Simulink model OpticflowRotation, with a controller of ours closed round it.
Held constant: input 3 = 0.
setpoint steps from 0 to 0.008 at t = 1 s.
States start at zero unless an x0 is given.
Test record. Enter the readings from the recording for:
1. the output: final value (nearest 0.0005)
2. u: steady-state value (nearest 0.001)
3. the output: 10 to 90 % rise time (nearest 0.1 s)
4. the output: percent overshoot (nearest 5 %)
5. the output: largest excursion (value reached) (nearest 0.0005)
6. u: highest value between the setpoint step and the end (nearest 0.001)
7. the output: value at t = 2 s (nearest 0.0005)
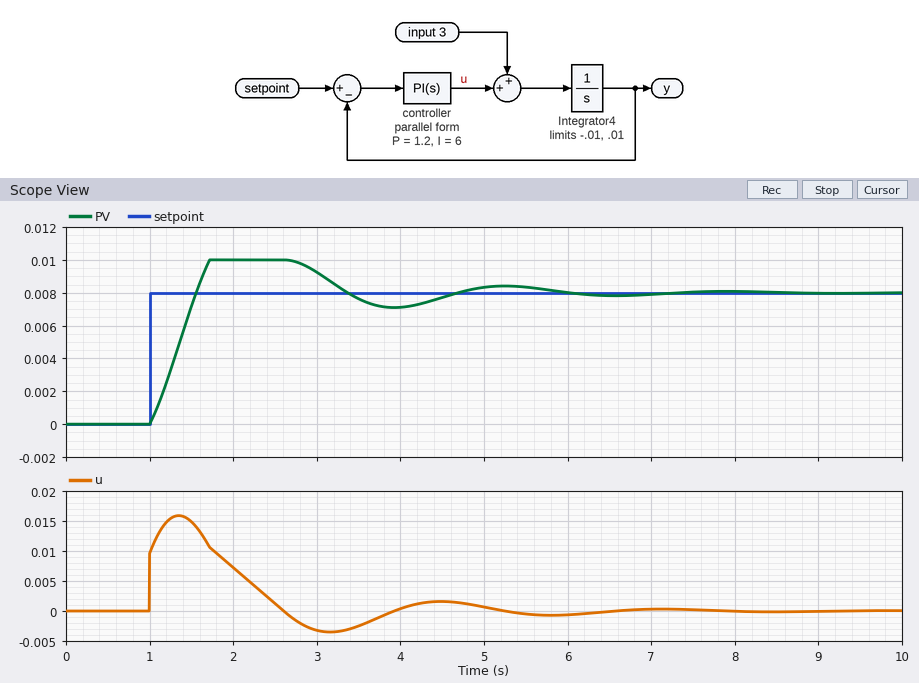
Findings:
0.0080
0.000
0.4 s
25 %
0.0100
0.016
0.0100
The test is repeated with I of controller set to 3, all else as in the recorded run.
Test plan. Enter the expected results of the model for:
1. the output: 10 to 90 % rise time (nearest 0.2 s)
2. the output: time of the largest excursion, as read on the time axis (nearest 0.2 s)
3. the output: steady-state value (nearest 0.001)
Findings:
0.6 s
2.0 s
0.008
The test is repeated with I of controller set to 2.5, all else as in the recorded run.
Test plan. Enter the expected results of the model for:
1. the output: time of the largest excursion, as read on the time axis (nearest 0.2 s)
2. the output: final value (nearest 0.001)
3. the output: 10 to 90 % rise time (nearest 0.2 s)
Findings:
2.2 s
0.008
0.6 s
